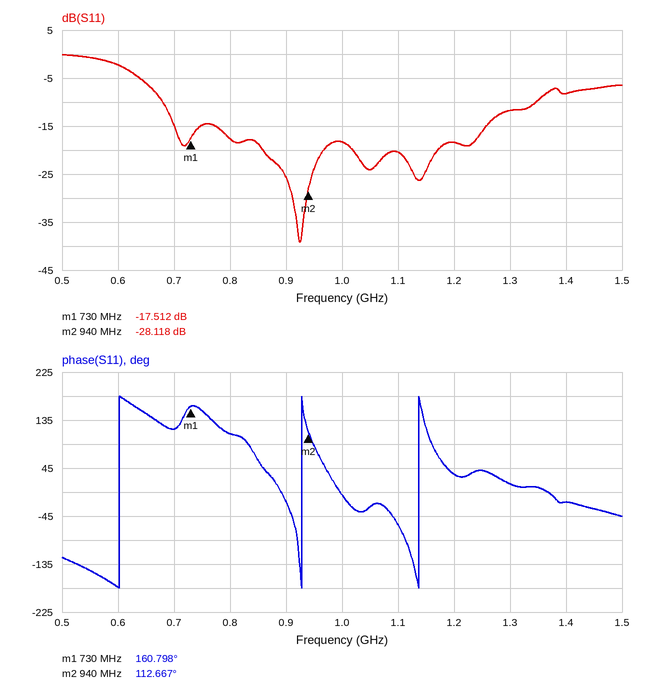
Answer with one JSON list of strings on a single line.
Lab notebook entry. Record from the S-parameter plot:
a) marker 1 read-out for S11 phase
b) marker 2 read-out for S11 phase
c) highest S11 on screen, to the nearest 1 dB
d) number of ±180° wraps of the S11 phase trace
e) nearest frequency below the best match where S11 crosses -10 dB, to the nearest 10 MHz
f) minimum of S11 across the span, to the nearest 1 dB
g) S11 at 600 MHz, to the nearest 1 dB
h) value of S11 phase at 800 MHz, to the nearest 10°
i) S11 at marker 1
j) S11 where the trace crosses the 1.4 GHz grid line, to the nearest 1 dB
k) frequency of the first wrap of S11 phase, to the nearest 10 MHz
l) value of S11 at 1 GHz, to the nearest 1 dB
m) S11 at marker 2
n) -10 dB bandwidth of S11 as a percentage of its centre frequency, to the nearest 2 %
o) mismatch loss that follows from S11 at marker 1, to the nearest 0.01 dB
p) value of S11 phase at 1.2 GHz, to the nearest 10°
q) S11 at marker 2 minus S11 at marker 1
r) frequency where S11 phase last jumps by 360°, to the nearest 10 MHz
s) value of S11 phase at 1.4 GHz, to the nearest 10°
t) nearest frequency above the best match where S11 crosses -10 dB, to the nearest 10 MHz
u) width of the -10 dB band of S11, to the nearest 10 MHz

["160.798°", "112.667°", "0 dB", "3", "680 MHz", "-39 dB", "-2 dB", "110°", "-17.512 dB", "-8 dB", "600 MHz", "-18 dB", "-28.118 dB", "66 %", "0.08 dB", "30°", "-10.606 dB", "1.14 GHz", "-20°", "1.35 GHz", "670 MHz"]
